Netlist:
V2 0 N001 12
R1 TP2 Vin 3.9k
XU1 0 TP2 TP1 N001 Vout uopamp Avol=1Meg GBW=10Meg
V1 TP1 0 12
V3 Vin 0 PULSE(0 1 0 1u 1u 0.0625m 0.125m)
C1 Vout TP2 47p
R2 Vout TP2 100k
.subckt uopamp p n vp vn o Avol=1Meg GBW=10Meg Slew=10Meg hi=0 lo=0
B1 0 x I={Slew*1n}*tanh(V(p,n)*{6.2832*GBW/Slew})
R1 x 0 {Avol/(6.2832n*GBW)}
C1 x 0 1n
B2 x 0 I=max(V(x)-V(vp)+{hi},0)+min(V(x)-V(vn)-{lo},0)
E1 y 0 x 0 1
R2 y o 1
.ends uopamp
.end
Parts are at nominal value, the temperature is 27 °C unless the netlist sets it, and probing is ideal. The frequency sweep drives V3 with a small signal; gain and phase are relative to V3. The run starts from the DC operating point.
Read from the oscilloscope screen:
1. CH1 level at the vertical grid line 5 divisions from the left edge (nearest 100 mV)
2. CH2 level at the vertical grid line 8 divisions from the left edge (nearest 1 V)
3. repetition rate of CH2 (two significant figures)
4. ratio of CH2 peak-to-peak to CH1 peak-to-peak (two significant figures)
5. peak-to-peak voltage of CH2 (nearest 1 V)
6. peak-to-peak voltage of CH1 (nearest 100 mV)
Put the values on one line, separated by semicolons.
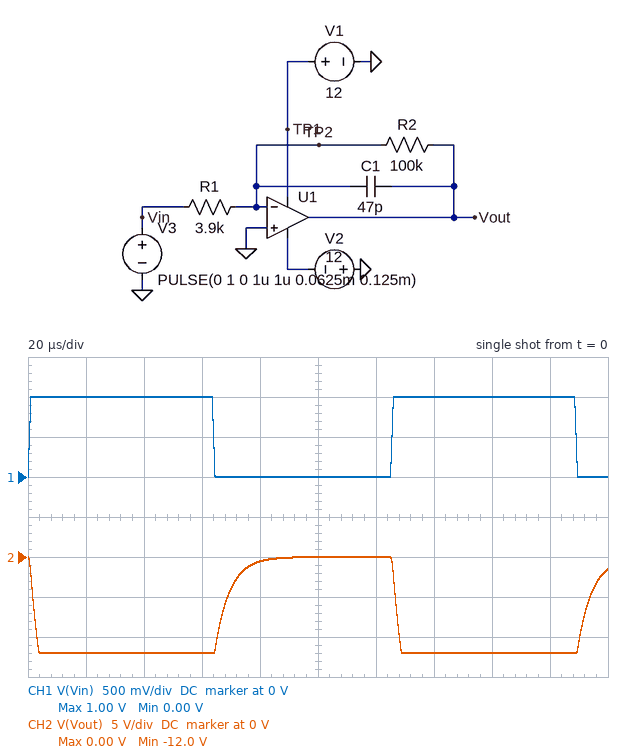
0 V; -12 V; 8.0 kHz; 12; 12 V; 1.0 V
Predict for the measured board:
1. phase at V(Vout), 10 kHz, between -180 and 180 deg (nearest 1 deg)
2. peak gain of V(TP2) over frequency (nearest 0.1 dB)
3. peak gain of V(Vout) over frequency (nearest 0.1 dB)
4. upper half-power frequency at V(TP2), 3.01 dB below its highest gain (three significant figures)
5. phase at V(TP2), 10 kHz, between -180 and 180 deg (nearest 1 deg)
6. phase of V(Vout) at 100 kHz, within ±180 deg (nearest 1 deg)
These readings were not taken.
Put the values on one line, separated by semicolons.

162 deg; -22.0 dB; 28.2 dB; 10.9 MHz; 72 deg; 107 deg
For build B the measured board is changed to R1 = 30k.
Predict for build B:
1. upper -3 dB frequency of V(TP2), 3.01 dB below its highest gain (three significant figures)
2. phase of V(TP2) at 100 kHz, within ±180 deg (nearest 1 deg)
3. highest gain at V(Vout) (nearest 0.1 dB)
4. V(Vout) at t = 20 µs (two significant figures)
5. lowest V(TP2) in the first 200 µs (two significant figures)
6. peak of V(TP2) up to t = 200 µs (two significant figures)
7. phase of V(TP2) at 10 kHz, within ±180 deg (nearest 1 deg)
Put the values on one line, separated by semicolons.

10.2 MHz; 18 deg; 10.5 dB; -3.3 V; -10 mV; 10 mV; 73 deg
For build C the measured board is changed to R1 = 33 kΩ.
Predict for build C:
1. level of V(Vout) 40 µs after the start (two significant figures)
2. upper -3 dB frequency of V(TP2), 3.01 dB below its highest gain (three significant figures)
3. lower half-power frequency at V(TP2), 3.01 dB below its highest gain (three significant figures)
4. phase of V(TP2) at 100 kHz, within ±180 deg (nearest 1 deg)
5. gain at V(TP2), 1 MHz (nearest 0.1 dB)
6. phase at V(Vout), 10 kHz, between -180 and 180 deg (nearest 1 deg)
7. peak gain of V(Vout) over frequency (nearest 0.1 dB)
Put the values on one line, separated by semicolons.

-3.0 V; 10.2 MHz; 33.3 kHz; 18 deg; -39.9 dB; 163 deg; 9.6 dB
